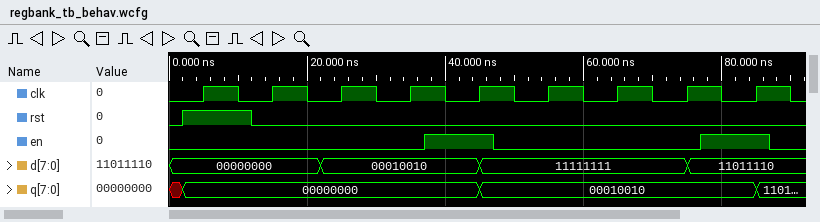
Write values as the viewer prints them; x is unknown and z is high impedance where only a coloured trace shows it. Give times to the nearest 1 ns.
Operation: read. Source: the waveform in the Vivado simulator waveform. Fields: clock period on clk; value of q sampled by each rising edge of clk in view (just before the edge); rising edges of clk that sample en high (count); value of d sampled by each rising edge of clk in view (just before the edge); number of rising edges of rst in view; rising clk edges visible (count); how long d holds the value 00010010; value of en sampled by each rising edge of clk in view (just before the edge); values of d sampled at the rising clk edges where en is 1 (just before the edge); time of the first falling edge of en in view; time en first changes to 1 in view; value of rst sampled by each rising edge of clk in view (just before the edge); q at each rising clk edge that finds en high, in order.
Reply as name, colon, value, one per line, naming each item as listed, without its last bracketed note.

clock period on clk: 10 ns
value of q sampled by each rising edge of clk in view: 00000000, 00000000, 00000000, 00000000, 00000000, 00010010, 00010010, 00010010, 00010010
rising edges of clk that sample en high: 2
value of d sampled by each rising edge of clk in view: 00000000, 00000000, 00010010, 00010010, 00010010, 11111111, 11111111, 11111111, 11011110
number of rising edges of rst in view: 1
rising clk edges visible: 9
how long d holds the value 00010010: 23 ns
value of en sampled by each rising edge of clk in view: 0 0 0 0 1 0 0 0 1
values of d sampled at the rising clk edges where en is 1: 00010010, 11011110
time of the first falling edge of en in view: 47 ns
time en first changes to 1 in view: 37 ns
value of rst sampled by each rising edge of clk in view: 1 0 0 0 0 0 0 0 0
q at each rising clk edge that finds en high, in order: 00000000, 00010010
